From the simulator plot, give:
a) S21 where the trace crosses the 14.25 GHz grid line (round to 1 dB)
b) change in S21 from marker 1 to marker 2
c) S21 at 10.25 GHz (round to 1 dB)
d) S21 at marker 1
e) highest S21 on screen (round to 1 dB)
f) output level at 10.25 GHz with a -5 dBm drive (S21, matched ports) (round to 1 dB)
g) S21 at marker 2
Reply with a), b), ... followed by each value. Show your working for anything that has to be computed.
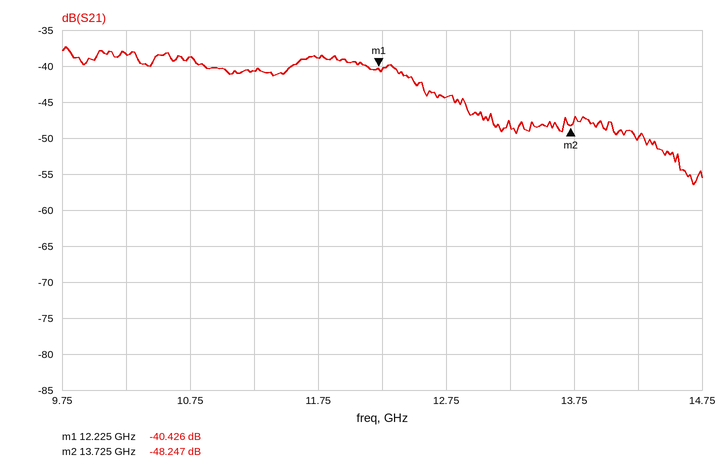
a) -50 dB
b) -48.247 − (-40.426) = -7.821 dB
c) -38 dB
d) -40.426 dB
e) -37 dB
f) -5 dBm + (-38 dB) = -43 dBm
g) -48.247 dB
